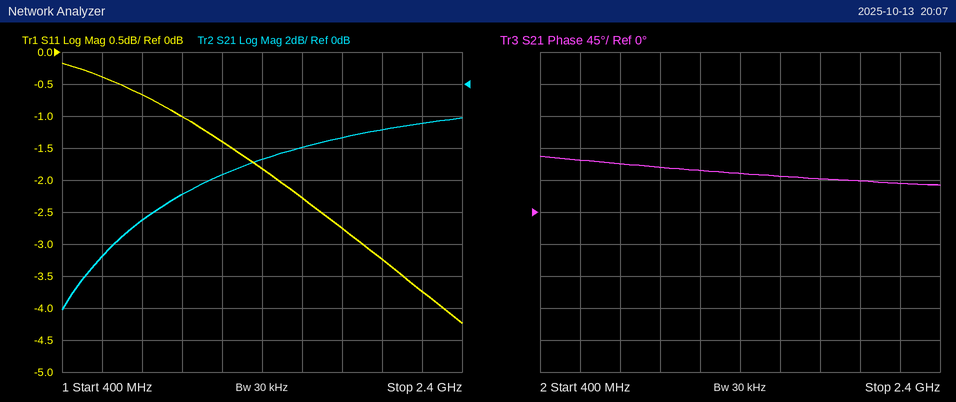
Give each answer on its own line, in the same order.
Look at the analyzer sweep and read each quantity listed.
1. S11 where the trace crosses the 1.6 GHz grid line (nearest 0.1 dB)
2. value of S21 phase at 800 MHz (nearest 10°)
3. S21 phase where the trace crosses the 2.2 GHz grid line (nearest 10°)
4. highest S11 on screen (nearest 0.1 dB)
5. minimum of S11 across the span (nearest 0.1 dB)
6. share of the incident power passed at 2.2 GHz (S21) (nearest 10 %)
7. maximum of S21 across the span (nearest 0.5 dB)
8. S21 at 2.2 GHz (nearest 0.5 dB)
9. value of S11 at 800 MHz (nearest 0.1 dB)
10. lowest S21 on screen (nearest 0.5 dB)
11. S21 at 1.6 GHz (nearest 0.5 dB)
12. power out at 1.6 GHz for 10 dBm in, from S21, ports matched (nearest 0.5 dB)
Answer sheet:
-2.3 dB
70°
40°
-0.2 dB
-4.2 dB
60 %
-2.0 dB
-2.5 dB
-0.7 dB
-14.0 dB
-4.0 dB
6.0 dBm
